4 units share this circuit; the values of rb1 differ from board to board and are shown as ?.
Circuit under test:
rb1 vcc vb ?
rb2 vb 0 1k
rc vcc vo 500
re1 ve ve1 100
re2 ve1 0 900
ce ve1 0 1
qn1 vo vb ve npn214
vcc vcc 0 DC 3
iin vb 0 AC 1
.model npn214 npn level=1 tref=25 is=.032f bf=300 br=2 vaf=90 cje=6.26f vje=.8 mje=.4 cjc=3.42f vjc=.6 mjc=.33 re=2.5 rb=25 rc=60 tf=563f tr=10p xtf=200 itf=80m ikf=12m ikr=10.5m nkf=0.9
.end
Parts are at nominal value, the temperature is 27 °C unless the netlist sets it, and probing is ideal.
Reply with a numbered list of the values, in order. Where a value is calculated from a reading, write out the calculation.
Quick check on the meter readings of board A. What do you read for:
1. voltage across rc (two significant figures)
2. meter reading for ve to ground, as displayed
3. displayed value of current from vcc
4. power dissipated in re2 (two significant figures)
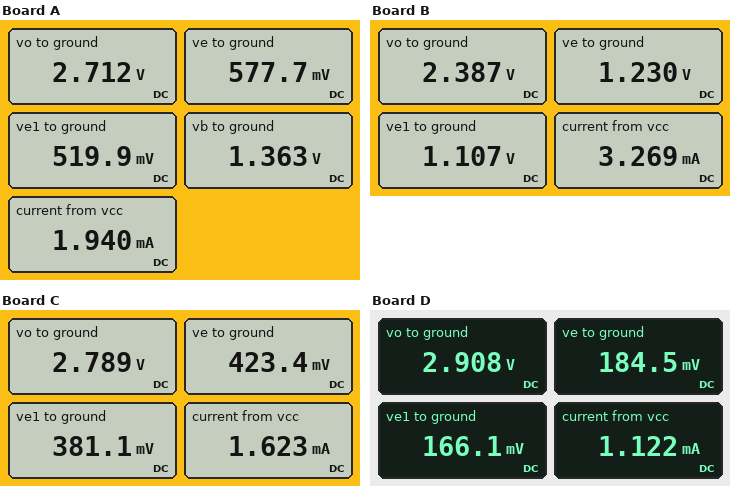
1. 3 V - 2.712 V = 290 mV
2. 577.7 mV
3. 1.940 mA
4. (519.9 mV)^2 / 900 Ω = 300 µW
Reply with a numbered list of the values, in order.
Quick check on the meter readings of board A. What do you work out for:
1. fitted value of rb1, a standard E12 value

1. 1.2 kΩ
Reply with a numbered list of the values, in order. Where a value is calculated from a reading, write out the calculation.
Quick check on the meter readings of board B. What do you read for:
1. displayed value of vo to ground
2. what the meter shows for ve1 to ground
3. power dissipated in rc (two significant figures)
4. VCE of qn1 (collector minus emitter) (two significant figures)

1. 2.387 V
2. 1.107 V
3. (3 V - 2.387 V)^2 / 500 Ω = 750 µW
4. 2.387 V - 1.23 V = 1.2 V
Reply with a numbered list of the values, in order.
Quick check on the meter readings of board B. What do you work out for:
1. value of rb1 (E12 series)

1. 470 Ω
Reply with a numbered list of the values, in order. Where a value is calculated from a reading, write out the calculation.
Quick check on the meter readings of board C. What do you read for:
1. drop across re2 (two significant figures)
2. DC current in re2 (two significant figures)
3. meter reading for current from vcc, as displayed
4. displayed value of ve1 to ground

1. 381.1 mV = 380 mV
2. (381.1 mV) / 900 Ω = 420 µA
3. 1.623 mA
4. 381.1 mV
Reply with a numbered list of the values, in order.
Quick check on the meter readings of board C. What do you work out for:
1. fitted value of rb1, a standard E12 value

1. 1.5 kΩ
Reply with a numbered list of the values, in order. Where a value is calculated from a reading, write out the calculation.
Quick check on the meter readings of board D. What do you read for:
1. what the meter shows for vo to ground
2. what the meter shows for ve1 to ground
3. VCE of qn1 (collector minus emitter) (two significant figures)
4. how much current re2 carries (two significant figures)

1. 2.908 V
2. 166.1 mV
3. 2.908 V - 184.5 mV = 2.7 V
4. (166.1 mV) / 900 Ω = 180 µA
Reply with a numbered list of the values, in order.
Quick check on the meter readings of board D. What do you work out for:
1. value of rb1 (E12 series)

1. 2.2 kΩ
